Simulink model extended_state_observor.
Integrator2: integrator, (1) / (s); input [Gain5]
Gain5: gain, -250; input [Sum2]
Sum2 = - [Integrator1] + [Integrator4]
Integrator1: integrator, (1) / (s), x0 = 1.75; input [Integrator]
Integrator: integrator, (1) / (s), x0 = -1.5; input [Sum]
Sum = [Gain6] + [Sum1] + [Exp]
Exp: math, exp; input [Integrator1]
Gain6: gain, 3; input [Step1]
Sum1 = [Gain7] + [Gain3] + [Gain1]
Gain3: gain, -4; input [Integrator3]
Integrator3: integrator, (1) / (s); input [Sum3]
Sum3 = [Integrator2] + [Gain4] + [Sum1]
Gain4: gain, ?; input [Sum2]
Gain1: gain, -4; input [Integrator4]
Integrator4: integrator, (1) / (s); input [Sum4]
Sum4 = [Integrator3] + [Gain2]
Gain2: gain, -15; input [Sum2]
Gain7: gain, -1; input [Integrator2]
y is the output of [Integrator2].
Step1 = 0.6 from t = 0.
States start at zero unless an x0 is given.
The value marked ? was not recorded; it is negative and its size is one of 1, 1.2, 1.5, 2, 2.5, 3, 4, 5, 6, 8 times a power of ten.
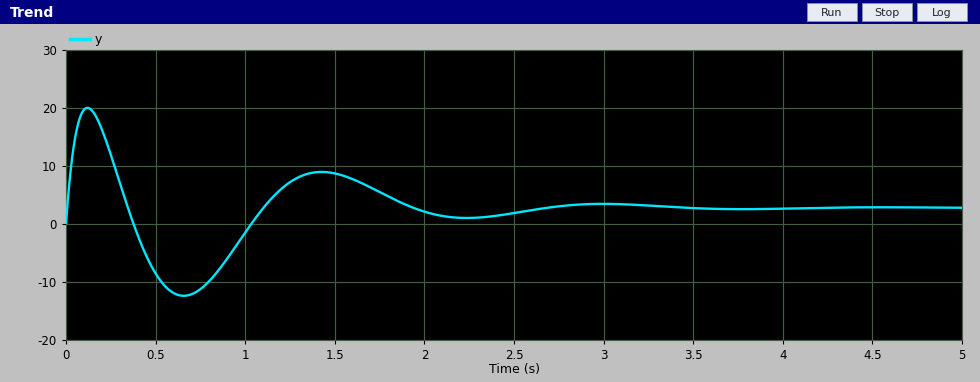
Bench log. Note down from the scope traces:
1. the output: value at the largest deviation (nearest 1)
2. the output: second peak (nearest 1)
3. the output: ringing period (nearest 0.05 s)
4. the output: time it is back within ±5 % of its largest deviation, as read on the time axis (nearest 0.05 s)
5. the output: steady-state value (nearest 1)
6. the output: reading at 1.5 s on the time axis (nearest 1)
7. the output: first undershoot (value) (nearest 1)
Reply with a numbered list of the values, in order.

1. 20
2. 9
3. 1.30 s
4. 2.50 s
5. 3
6. 9
7. -12
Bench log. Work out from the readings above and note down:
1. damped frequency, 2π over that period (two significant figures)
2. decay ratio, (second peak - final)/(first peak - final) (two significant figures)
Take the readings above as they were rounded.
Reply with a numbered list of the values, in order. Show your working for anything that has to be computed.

1. 2π / 1.3 = 4.8 rad/s
2. (9 - 3) / (20 - 3) = 0.35
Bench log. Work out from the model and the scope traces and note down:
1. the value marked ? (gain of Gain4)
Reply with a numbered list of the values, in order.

1. -50
